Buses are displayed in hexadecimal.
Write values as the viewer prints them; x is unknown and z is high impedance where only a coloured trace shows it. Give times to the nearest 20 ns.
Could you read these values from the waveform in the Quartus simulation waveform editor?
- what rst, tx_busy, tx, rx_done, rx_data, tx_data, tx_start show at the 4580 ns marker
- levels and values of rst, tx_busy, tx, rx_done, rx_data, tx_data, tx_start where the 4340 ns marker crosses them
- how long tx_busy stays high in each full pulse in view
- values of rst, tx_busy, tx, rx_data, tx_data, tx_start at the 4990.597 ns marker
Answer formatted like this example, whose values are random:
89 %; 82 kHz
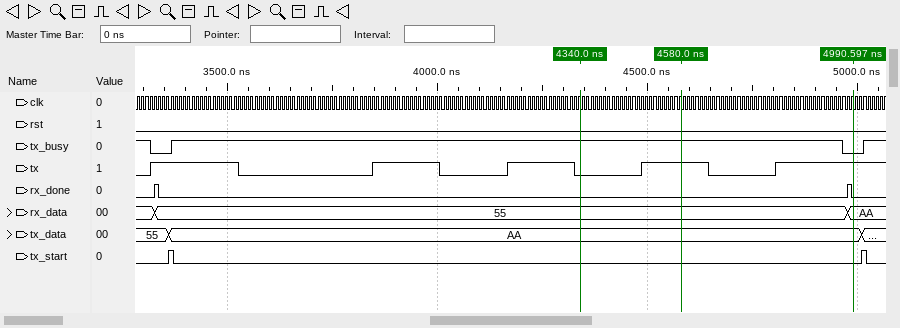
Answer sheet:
rst=0, tx_busy=1, tx=1, rx_done=0, rx_data=55, tx_data=AA, tx_start=0; rst=0, tx_busy=1, tx=0, rx_done=0, rx_data=55, tx_data=AA, tx_start=0; 1600 ns; rst=0, tx_busy=0, tx=1, rx_data=AA, tx_data=AA, tx_start=0
